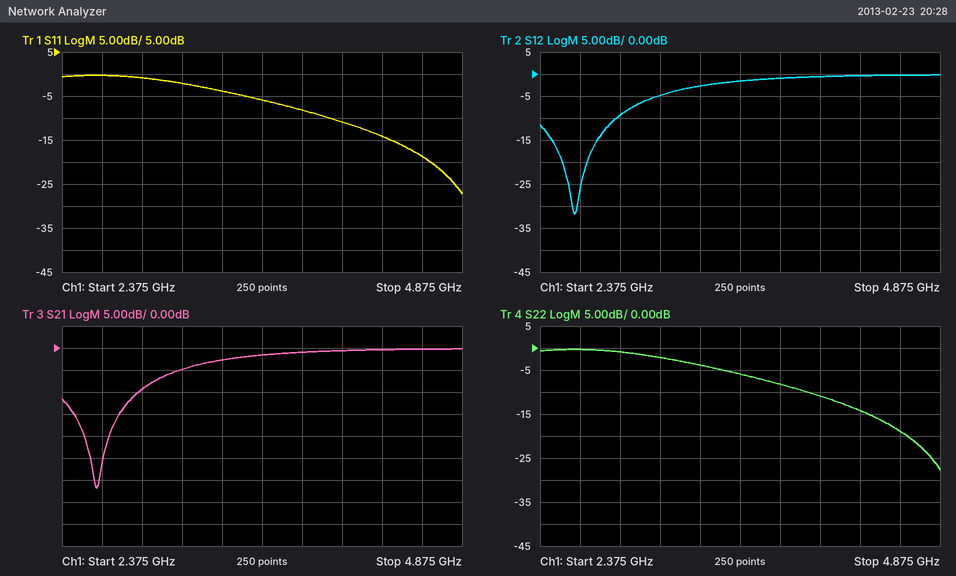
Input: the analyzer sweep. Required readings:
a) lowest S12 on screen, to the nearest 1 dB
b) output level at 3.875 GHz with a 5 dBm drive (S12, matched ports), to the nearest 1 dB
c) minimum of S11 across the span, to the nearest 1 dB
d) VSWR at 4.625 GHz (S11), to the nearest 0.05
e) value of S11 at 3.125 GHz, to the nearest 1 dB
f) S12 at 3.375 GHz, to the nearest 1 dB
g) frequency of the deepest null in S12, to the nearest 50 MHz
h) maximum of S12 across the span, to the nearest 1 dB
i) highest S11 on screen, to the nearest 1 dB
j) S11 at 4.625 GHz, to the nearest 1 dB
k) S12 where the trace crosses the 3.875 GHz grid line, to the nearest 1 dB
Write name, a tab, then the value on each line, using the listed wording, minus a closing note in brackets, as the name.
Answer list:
lowest S12 on screen, to the nearest 1 dB	-32 dB
output level at 3.875 GHz with a 5 dBm drive (S12, matched ports), to the nearest 1 dB	4 dBm
minimum of S11 across the span, to the nearest 1 dB	-27 dB
VSWR at 4.625 GHz (S11), to the nearest 0.05	1.25
value of S11 at 3.125 GHz, to the nearest 1 dB	-2 dB
S12 at 3.375 GHz, to the nearest 1 dB	-3 dB
frequency of the deepest null in S12, to the nearest 50 MHz	2.60 GHz
maximum of S12 across the span, to the nearest 1 dB	0 dB
highest S11 on screen, to the nearest 1 dB	0 dB
S11 at 4.625 GHz, to the nearest 1 dB	-19 dB
S12 where the trace crosses the 3.875 GHz grid line, to the nearest 1 dB	-1 dB
